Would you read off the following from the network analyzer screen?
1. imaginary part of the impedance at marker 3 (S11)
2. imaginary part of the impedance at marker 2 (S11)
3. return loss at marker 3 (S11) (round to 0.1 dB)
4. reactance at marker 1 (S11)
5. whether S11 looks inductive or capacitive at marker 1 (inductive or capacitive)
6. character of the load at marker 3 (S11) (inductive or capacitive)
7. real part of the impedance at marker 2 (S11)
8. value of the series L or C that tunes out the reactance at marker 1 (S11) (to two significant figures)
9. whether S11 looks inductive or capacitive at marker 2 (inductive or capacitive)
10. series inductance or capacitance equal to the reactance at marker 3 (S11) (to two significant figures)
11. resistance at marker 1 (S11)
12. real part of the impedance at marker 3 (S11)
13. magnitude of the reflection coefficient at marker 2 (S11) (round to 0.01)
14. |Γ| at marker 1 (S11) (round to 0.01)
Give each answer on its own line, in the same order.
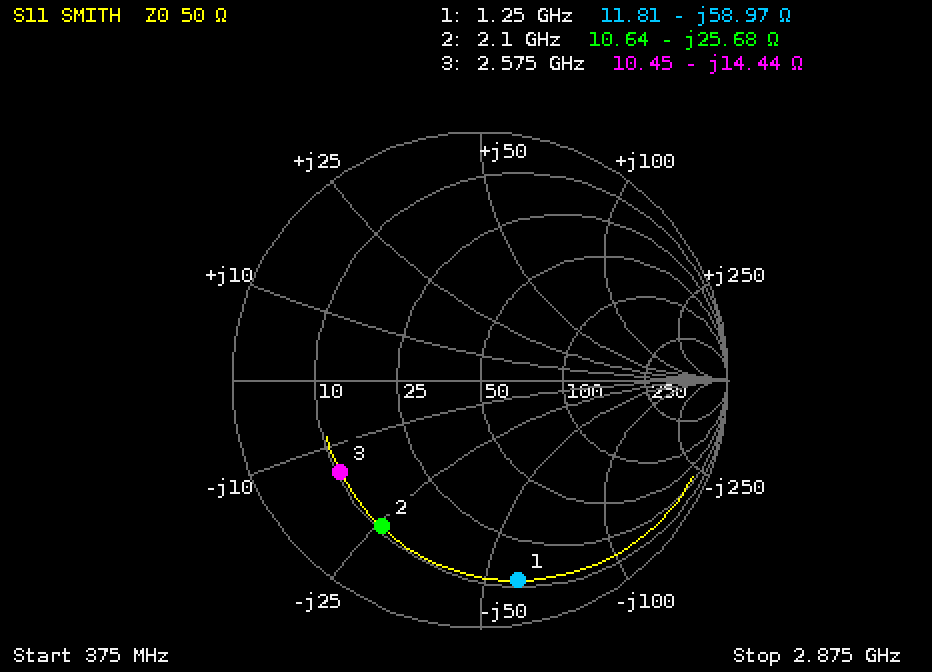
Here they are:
-14.44 Ω
-25.68 Ω
3.4 dB
-58.97 Ω
capacitive
capacitive
10.64 Ω
7.5 nH
capacitive
4.3 pF
11.81 Ω
10.45 Ω
0.71
0.82
